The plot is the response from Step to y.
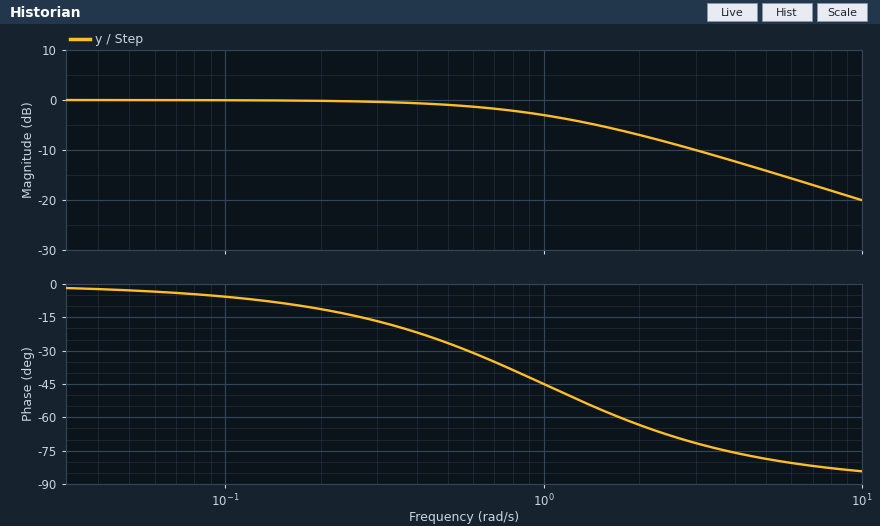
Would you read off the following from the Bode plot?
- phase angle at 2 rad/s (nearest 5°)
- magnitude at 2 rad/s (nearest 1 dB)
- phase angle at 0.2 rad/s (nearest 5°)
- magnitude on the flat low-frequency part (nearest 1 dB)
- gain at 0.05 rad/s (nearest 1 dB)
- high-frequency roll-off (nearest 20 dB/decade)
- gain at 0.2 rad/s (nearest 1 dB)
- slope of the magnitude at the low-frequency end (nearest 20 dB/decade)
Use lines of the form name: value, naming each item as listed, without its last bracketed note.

phase angle at 2 rad/s: -65°
magnitude at 2 rad/s: -7 dB
phase angle at 0.2 rad/s: -10°
magnitude on the flat low-frequency part: 0 dB
gain at 0.05 rad/s: 0 dB
high-frequency roll-off: -20 dB/decade
gain at 0.2 rad/s: 0 dB
slope of the magnitude at the low-frequency end: 0 dB/decade
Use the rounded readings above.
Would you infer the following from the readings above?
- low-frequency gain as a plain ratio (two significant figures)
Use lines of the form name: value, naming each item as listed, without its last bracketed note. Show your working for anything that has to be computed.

low-frequency gain as a plain ratio: 10^(0 / 20) = 1.0
